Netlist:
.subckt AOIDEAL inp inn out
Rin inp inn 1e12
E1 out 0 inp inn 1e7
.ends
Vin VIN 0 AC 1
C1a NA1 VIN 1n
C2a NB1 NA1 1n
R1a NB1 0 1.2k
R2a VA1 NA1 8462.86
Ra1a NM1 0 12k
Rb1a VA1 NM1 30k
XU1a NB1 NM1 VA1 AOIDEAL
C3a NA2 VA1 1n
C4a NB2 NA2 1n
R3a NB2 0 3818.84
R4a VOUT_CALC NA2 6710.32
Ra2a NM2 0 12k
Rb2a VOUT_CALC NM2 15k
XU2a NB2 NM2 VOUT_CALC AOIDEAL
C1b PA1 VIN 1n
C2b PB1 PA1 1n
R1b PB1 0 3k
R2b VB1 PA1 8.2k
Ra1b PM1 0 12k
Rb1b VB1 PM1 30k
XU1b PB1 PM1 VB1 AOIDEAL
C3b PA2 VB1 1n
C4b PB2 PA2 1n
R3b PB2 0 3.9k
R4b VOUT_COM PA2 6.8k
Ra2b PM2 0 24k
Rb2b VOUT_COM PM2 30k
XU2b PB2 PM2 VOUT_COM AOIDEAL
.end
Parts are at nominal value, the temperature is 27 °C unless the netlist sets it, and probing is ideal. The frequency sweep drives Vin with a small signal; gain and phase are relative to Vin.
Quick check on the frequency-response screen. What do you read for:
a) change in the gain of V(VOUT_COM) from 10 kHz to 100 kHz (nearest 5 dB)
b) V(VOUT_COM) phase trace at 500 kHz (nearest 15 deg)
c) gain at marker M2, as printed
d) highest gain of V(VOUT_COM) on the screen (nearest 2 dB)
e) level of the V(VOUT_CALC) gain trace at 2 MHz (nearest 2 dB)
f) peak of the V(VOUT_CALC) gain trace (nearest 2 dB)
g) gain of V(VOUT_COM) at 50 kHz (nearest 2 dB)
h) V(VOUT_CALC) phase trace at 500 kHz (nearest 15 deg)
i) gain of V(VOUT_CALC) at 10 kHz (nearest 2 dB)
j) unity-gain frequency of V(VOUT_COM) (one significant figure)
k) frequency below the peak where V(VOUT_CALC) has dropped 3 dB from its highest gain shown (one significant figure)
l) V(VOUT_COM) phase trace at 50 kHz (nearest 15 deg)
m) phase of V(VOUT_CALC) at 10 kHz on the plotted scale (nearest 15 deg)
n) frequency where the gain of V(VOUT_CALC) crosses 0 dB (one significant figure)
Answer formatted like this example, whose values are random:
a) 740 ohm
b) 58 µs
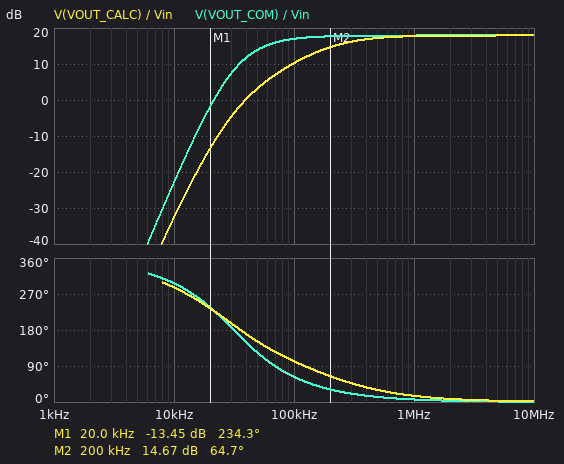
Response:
a) 40 dB
b) 15 deg
c) 14.67 dB
d) 18 dB
e) 18 dB
f) 18 dB
g) 14 dB
h) 30 deg
i) -32 dB
j) 20 kHz
k) 200 kHz
l) 120 deg
m) 285 deg
n) 40 kHz
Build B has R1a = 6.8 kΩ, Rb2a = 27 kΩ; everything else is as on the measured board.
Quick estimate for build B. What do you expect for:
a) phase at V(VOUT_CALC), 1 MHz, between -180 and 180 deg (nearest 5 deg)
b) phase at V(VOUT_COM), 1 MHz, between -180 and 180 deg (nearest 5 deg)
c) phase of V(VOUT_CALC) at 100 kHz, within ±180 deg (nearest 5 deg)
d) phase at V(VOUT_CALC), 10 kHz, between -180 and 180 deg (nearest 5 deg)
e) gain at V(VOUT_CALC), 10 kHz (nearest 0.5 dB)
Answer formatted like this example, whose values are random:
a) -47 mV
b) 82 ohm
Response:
a) 0 deg
b) 5 deg
c) 20 deg
d) -20 deg
e) -9.0 dB
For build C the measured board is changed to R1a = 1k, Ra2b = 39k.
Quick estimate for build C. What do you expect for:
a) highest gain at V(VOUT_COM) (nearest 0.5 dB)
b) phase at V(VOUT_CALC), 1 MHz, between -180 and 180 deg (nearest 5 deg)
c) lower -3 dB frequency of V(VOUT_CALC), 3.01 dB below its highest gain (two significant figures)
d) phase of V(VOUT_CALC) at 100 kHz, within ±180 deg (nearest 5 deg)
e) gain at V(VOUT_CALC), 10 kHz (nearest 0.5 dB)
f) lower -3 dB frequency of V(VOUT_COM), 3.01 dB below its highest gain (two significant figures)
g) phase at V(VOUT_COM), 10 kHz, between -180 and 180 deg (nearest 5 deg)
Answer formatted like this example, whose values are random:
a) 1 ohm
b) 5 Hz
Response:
a) 16.0 dB
b) 20 deg
c) 260 kHz
d) 105 deg
e) -34.5 dB
f) 68 kHz
g) -70 deg
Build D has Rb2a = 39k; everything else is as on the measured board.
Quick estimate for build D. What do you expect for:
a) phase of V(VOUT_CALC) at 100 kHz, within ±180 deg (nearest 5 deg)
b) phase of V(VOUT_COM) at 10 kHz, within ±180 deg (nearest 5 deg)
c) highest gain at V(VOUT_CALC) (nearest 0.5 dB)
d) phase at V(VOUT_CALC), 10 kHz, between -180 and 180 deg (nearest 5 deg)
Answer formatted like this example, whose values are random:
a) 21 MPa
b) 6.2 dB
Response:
a) 75 deg
b) -65 deg
c) 23.5 dB
d) -45 deg
